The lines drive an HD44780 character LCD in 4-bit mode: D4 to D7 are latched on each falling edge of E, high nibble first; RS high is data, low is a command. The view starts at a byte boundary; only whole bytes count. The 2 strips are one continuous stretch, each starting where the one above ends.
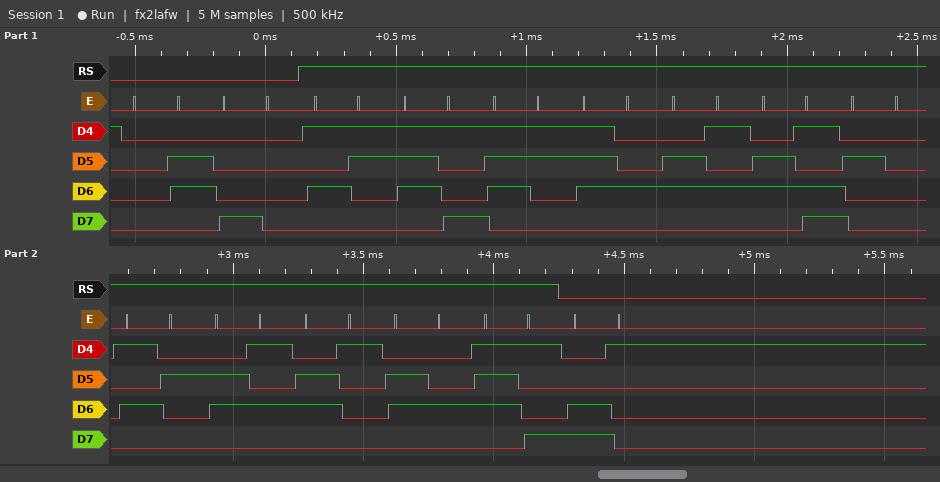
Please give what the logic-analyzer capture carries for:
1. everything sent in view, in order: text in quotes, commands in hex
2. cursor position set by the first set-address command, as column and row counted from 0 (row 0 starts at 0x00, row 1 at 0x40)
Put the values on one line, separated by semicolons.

0x06 0x80 "System Ready" 0xC1; column 0, row 0
